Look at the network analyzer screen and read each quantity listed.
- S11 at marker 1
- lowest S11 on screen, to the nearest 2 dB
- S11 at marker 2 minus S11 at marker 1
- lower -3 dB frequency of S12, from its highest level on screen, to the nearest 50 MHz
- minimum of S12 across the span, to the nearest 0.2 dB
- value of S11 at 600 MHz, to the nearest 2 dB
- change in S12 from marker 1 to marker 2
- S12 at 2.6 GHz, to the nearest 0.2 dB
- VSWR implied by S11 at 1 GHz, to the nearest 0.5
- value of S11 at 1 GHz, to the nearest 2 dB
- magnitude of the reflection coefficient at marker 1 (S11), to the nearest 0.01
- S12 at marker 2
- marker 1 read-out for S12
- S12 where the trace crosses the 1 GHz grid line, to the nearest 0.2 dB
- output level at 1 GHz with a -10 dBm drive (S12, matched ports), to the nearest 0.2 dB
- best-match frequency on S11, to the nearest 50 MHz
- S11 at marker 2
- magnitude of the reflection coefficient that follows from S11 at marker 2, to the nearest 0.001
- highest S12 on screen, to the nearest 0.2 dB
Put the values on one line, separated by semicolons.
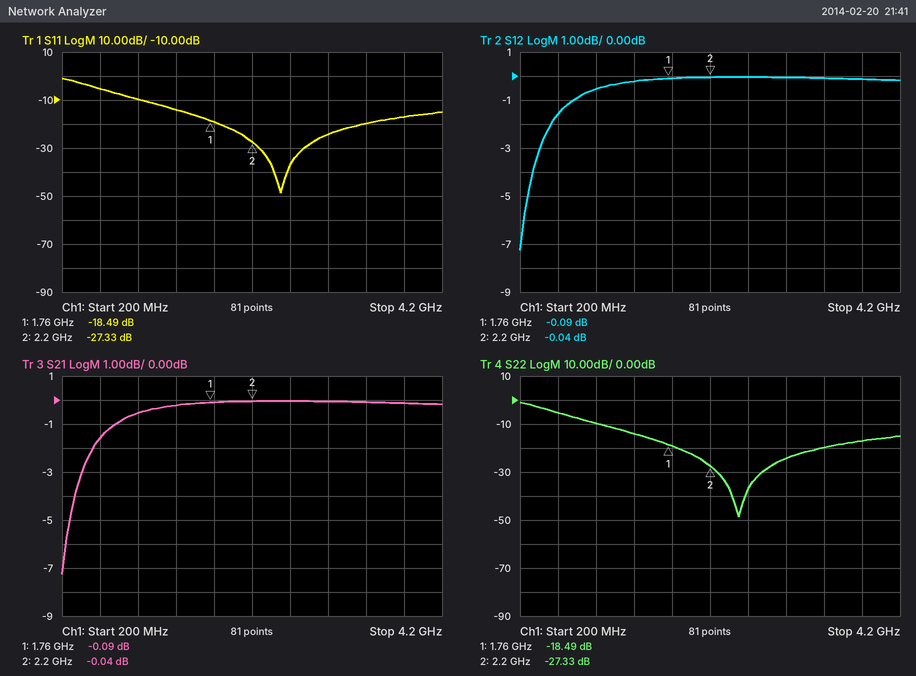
-18.49 dB; -48 dB; -8.84 dB; 400 MHz; -7.2 dB; -6 dB; 0.05 dB; 0.0 dB; 2.0; -10 dB; 0.12; -0.04 dB; -0.09 dB; -0.6 dB; -10.6 dBm; 2.50 GHz; -27.33 dB; 0.043; 0.0 dB
